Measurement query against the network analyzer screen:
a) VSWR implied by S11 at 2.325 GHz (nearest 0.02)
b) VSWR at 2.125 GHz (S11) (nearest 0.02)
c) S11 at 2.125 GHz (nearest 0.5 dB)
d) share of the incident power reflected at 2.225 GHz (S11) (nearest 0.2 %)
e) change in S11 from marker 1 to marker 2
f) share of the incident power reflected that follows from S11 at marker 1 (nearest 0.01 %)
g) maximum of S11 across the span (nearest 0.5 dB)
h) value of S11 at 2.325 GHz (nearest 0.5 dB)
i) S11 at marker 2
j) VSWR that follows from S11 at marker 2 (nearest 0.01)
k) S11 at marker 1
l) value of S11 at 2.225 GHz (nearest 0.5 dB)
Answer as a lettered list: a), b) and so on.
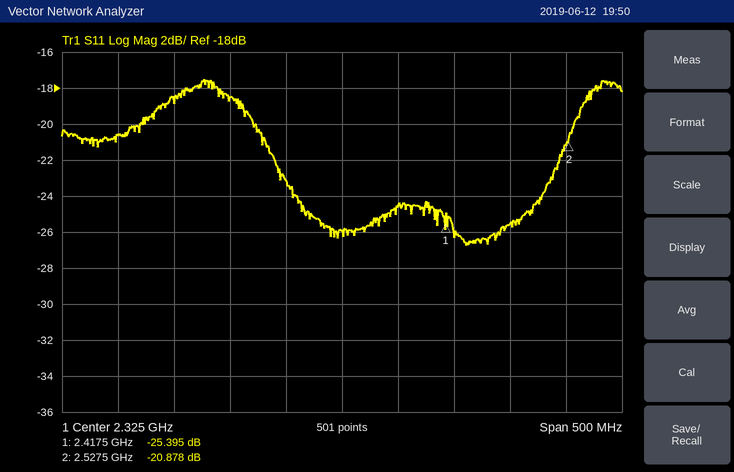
a) 1.10
b) 1.20
c) -20.5 dB
d) 1.4 %
e) 4.517 dB
f) 0.29 %
g) -17.5 dB
h) -26.0 dB
i) -20.878 dB
j) 1.20
k) -25.395 dB
l) -18.5 dB
